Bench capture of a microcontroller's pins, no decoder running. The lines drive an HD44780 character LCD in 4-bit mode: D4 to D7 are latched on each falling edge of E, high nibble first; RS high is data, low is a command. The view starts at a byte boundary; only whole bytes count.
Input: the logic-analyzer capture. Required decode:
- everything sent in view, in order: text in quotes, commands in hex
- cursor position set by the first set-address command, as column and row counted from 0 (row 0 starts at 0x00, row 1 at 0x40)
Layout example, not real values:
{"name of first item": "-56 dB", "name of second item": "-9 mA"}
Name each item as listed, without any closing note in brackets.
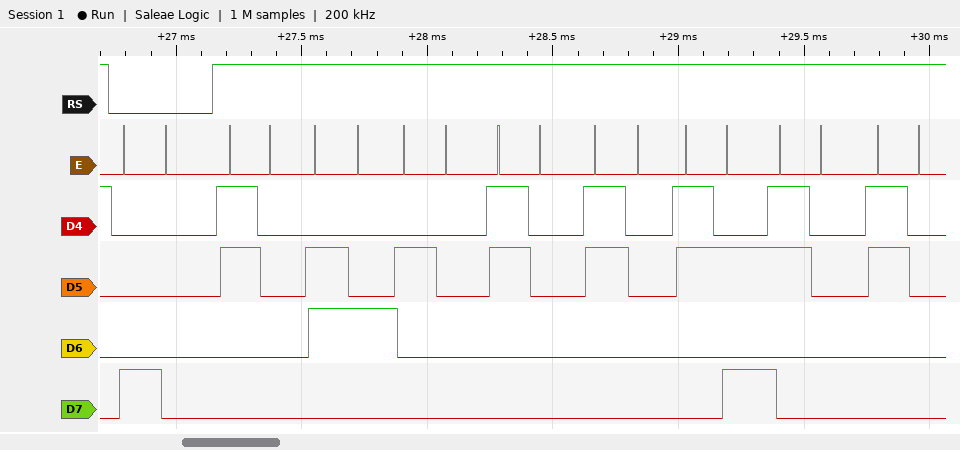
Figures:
{"everything sent in view, in order: text in quotes, commands in hex": "0x80 \"0d 00:00\"", "cursor position set by the first set-address command, as column and row counted from 0": "column 0, row 0"}
